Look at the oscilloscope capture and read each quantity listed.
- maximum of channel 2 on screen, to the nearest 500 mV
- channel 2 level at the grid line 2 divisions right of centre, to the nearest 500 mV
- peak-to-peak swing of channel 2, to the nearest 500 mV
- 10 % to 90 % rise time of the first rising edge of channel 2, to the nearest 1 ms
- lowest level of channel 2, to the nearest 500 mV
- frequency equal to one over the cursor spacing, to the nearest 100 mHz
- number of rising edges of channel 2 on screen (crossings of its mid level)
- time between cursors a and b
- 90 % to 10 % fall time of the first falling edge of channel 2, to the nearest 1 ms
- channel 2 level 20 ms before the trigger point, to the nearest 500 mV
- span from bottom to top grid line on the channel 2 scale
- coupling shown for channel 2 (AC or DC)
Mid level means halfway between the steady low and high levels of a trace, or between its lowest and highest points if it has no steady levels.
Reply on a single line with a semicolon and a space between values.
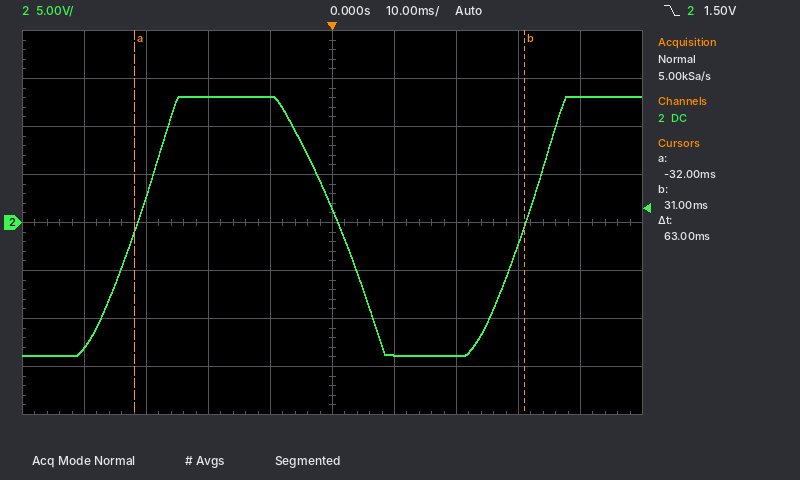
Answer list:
13.0 V; -14.0 V; 27.0 V; 12 ms; -14.0 V; 15.9 Hz; 2; 63 ms; 14 ms; 13.0 V; 40 V; DC
